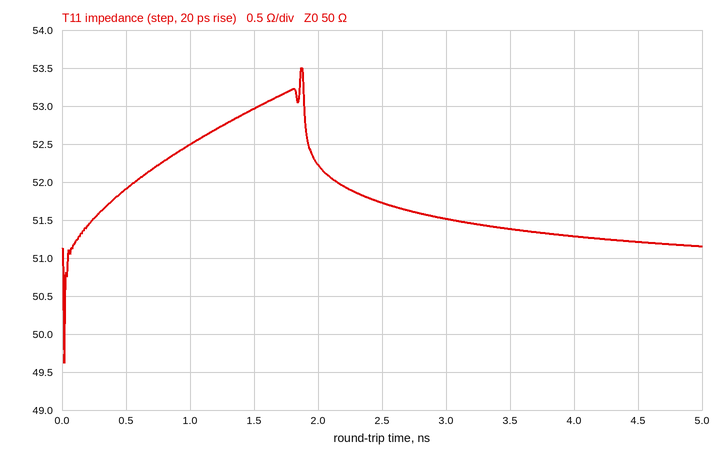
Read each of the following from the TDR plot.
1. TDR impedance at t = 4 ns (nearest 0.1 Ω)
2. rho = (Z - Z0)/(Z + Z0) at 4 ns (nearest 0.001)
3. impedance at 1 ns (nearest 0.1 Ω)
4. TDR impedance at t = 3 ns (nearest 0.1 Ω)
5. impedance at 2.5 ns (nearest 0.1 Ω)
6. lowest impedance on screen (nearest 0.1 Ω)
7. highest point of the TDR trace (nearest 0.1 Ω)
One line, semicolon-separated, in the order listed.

51.3 Ω; +0.013; 52.5 Ω; 51.5 Ω; 51.7 Ω; 49.6 Ω; 53.5 Ω
